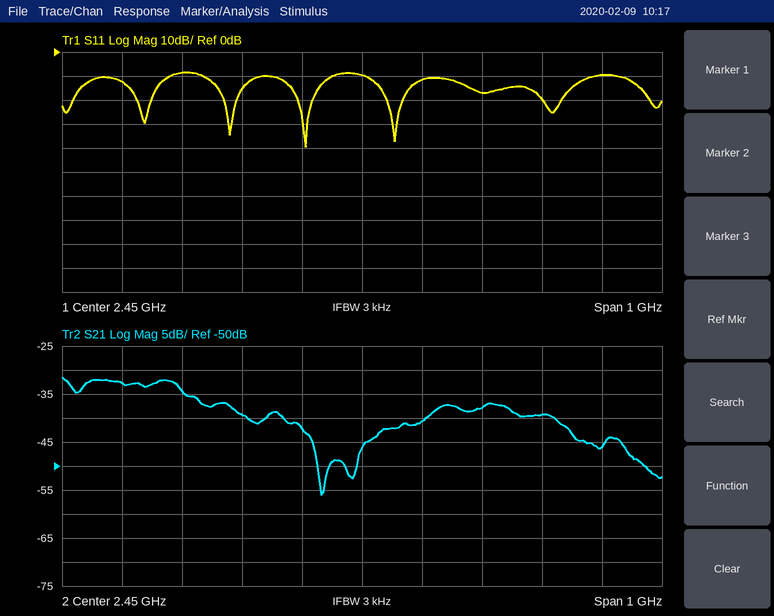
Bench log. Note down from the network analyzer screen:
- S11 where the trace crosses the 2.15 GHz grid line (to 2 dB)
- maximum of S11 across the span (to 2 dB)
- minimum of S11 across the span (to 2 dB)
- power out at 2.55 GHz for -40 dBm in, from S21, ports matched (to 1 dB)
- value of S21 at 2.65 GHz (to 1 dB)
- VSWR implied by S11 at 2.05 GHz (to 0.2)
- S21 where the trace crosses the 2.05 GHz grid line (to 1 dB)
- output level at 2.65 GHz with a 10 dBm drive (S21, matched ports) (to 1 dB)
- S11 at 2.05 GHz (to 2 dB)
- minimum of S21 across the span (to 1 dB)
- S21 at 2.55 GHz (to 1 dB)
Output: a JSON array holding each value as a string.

["-8 dB", "-8 dB", "-40 dB", "-81 dBm", "-38 dB", "1.6", "-33 dB", "-28 dBm", "-12 dB", "-56 dB", "-41 dB"]
